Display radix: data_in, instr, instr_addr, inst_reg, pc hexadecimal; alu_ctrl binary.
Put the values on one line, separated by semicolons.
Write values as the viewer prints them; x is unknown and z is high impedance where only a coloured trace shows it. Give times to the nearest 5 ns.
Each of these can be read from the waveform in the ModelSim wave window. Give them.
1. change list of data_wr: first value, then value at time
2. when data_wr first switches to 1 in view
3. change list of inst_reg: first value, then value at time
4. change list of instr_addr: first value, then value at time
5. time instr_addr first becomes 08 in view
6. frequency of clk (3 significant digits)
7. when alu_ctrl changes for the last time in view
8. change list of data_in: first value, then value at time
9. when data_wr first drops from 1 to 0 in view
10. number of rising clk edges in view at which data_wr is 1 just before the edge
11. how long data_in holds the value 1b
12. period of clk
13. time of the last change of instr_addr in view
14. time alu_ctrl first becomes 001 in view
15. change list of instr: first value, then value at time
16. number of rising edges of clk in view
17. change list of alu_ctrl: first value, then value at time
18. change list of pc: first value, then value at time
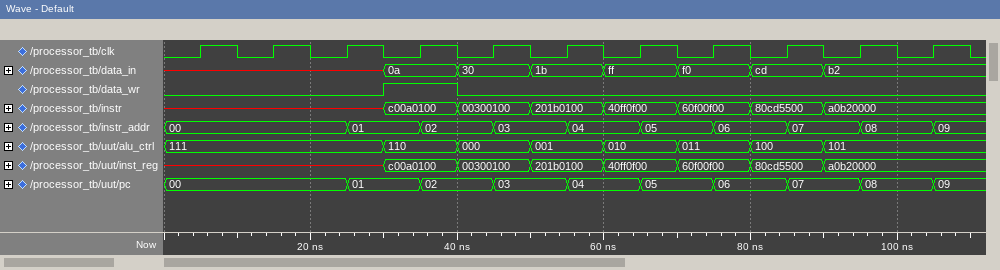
0, 1 at 30 ns, 0 at 40 ns; 30 ns; x, c00a0100 at 30 ns, 00300100 at 40 ns, 201b0100 at 50 ns, 40ff0f00 at 60 ns, 60f00f00 at 70 ns, 80cd5500 at 80 ns, a0b20000 at 90 ns; 00, 01 at 25 ns, 02 at 35 ns, 03 at 45 ns, 04 at 55 ns, 05 at 65 ns, 06 at 75 ns, 07 at 85 ns, 08 at 95 ns, 09 at 105 ns; 95 ns; 100 MHz; 90 ns; x, 0a at 30 ns, 30 at 40 ns, 1b at 50 ns, ff at 60 ns, f0 at 70 ns, cd at 80 ns, b2 at 90 ns; 40 ns; 1; 10 ns; 10 ns; 105 ns; 50 ns; x, c00a0100 at 30 ns, 00300100 at 40 ns, 201b0100 at 50 ns, 40ff0f00 at 60 ns, 60f00f00 at 70 ns, 80cd5500 at 80 ns, a0b20000 at 90 ns; 11; 111, 110 at 30 ns, 000 at 40 ns, 001 at 50 ns, 010 at 60 ns, 011 at 70 ns, 100 at 80 ns, 101 at 90 ns; 00, 01 at 25 ns, 02 at 35 ns, 03 at 45 ns, 04 at 55 ns, 05 at 65 ns, 06 at 75 ns, 07 at 85 ns, 08 at 95 ns, 09 at 105 ns
